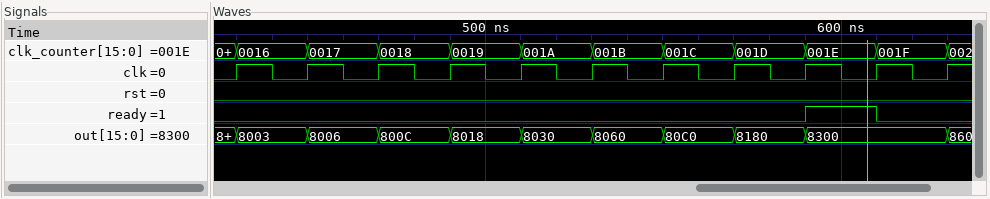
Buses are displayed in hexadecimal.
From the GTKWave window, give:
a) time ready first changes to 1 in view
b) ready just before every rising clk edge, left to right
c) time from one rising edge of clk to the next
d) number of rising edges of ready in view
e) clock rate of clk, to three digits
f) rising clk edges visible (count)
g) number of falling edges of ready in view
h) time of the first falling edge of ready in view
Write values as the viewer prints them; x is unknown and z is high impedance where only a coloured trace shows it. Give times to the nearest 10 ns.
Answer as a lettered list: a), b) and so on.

a) 590 ns
b) 0 0 0 0 0 0 0 0 0 1 0
c) 20 ns
d) 1
e) 50.0 MHz
f) 11
g) 1
h) 610 ns
